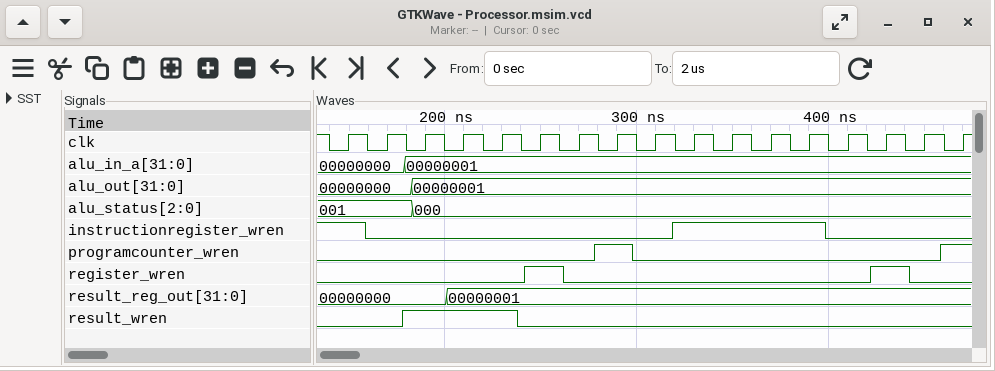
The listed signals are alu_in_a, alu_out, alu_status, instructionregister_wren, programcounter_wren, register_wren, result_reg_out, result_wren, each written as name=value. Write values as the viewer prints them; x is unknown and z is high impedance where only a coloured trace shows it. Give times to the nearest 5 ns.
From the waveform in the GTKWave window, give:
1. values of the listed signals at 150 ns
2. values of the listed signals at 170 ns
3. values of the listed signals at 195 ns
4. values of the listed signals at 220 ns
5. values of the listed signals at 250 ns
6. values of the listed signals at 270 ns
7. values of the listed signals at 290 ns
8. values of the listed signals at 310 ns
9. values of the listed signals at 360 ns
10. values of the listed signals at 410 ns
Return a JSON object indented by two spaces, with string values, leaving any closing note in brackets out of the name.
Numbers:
{
  "values of the listed signals at 150 ns": "alu_in_a=00000000, alu_out=00000000, alu_status=001, instructionregister_wren=1, programcounter_wren=0, register_wren=0, result_reg_out=00000000, result_wren=0",
  "values of the listed signals at 170 ns": "alu_in_a=00000000, alu_out=00000000, alu_status=001, instructionregister_wren=0, programcounter_wren=0, register_wren=0, result_reg_out=00000000, result_wren=0",
  "values of the listed signals at 195 ns": "alu_in_a=00000001, alu_out=00000001, alu_status=000, instructionregister_wren=0, programcounter_wren=0, register_wren=0, result_reg_out=00000000, result_wren=1",
  "values of the listed signals at 220 ns": "alu_in_a=00000001, alu_out=00000001, alu_status=000, instructionregister_wren=0, programcounter_wren=0, register_wren=0, result_reg_out=00000001, result_wren=1",
  "values of the listed signals at 250 ns": "alu_in_a=00000001, alu_out=00000001, alu_status=000, instructionregister_wren=0, programcounter_wren=0, register_wren=1, result_reg_out=00000001, result_wren=0",
  "values of the listed signals at 270 ns": "alu_in_a=00000001, alu_out=00000001, alu_status=000, instructionregister_wren=0, programcounter_wren=0, register_wren=0, result_reg_out=00000001, result_wren=0",
  "values of the listed signals at 290 ns": "alu_in_a=00000001, alu_out=00000001, alu_status=000, instructionregister_wren=0, programcounter_wren=1, register_wren=0, result_reg_out=00000001, result_wren=0",
  "values of the listed signals at 310 ns": "alu_in_a=00000001, alu_out=00000001, alu_status=000, instructionregister_wren=0, programcounter_wren=0, register_wren=0, result_reg_out=00000001, result_wren=0",
  "values of the listed signals at 360 ns": "alu_in_a=00000001, alu_out=00000001, alu_status=000, instructionregister_wren=1, programcounter_wren=0, register_wren=0, result_reg_out=00000001, result_wren=0",
  "values of the listed signals at 410 ns": "alu_in_a=00000001, alu_out=00000001, alu_status=000, instructionregister_wren=0, programcounter_wren=0, register_wren=0, result_reg_out=00000001, result_wren=0"
}
